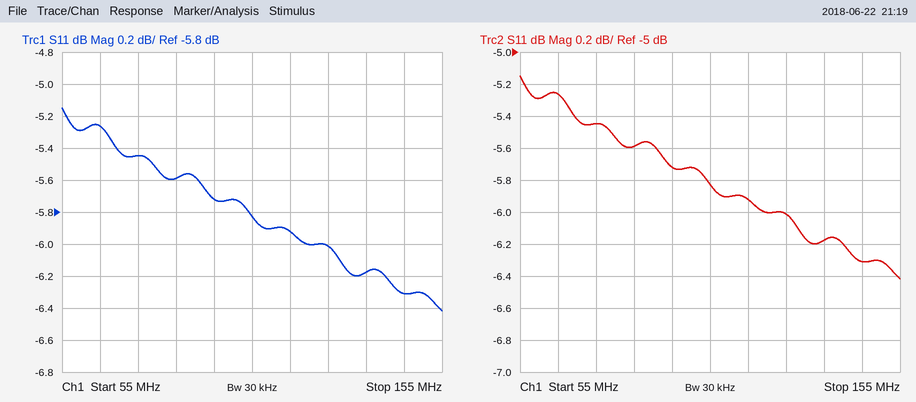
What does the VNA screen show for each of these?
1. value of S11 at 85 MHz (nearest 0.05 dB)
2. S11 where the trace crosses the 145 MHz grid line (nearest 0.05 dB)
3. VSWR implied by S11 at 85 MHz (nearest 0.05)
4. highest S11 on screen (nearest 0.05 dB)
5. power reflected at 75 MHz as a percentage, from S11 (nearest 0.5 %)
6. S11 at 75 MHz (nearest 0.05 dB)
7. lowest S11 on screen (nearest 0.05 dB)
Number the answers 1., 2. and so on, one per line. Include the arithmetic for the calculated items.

1. -5.60 dB
2. -6.30 dB
3. |Γ| = 10^(-5.6/20) = 0.5248; VSWR = (1 + 0.5248)/(1 − 0.5248) ≈ 3.21, so 3.20 to the nearest 0.05
4. -5.15 dB
5. 10^(-5.45/10) ≈ 28.5 %
6. -5.45 dB
7. -6.40 dB
